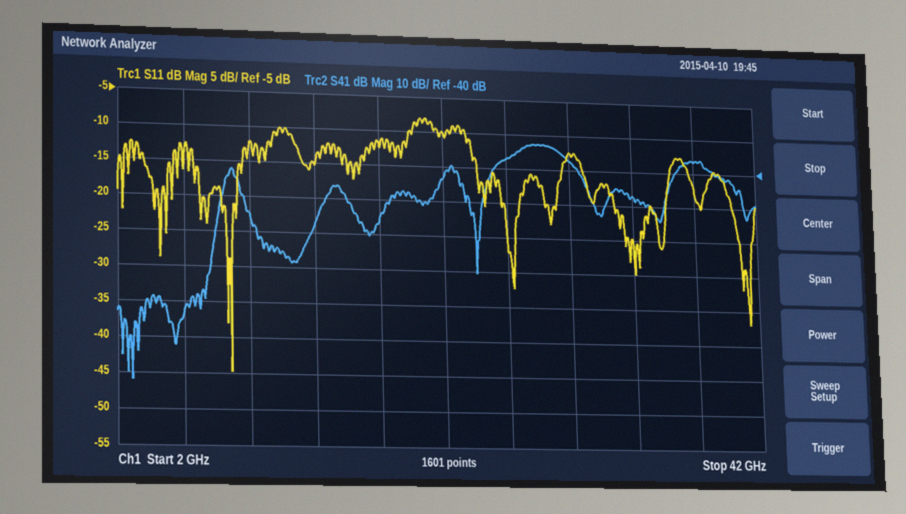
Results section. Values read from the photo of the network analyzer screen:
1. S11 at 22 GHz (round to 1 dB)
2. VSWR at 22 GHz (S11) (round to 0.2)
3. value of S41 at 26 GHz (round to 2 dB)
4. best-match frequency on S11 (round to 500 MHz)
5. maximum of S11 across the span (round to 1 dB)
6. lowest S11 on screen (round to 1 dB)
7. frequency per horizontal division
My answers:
-10 dB
2.0
-38 dB
9.0 GHz
-8 dB
-45 dB
4 GHz
